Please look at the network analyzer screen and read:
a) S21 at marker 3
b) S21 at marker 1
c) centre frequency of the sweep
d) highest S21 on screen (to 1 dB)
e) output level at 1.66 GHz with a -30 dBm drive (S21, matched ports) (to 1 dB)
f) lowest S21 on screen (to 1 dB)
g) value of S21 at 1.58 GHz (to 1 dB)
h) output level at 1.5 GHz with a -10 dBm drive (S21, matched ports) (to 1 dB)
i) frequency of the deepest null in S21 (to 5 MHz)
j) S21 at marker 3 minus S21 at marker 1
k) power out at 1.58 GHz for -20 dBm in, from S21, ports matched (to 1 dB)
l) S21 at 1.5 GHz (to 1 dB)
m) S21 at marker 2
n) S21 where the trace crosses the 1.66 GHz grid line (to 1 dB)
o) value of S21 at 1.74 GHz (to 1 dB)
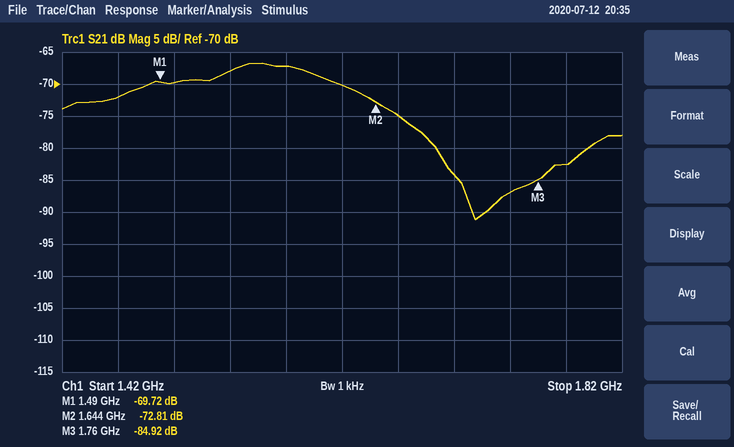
-84.92 dB
-69.72 dB
1.62 GHz
-67 dB
-105 dBm
-91 dB
-67 dB
-80 dBm
1.715 GHz
-15.20 dB
-87 dBm
-70 dB
-72.81 dB
-75 dB
-87 dB
